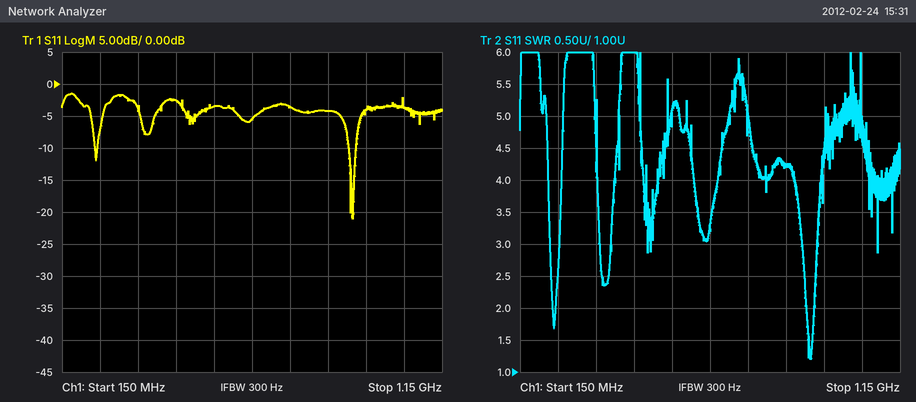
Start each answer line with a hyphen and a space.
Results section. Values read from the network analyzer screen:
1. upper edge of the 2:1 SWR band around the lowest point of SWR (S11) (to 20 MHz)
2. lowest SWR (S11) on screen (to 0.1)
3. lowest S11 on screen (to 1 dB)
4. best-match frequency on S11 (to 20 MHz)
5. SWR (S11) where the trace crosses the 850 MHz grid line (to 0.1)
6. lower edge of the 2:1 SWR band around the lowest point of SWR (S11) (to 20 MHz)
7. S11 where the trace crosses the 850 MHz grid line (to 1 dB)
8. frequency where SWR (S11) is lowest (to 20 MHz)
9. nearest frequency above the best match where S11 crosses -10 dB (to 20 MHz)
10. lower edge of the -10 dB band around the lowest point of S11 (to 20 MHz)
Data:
- 920 MHz
- 1.2
- -21 dB
- 920 MHz
- 4.2
- 900 MHz
- -4 dB
- 920 MHz
- 920 MHz
- 900 MHz
